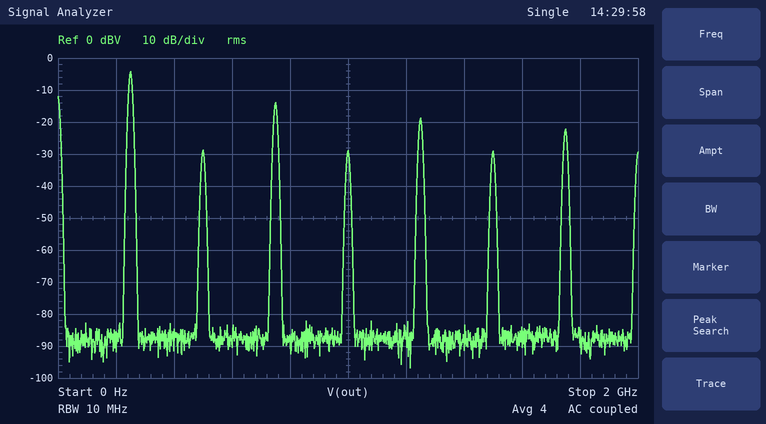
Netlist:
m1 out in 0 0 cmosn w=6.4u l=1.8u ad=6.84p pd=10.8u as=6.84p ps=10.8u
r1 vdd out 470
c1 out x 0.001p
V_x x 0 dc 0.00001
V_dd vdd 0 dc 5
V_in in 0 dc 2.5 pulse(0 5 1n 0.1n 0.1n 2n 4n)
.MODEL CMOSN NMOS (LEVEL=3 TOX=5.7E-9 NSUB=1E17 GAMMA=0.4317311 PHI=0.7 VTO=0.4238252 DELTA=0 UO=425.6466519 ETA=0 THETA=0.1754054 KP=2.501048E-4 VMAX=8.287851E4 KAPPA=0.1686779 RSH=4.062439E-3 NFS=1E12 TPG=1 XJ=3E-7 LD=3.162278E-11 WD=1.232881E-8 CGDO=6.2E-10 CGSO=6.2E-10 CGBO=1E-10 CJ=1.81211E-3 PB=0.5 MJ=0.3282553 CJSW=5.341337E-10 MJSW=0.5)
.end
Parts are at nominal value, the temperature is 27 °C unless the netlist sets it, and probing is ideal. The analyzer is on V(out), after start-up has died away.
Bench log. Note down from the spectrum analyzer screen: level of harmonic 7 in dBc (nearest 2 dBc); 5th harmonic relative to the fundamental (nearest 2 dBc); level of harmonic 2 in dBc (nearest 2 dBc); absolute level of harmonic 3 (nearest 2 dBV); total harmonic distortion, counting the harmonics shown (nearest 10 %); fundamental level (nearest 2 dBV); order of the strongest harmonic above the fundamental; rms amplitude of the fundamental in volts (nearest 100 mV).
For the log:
-18 dBc
-14 dBc
-24 dBc
-14 dBV
40 %
-4 dBV
3
600 mV
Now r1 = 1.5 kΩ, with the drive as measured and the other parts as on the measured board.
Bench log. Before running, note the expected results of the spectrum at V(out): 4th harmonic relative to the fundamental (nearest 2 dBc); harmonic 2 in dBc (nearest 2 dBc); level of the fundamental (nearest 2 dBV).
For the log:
-22 dBc
-22 dBc
4 dBV
